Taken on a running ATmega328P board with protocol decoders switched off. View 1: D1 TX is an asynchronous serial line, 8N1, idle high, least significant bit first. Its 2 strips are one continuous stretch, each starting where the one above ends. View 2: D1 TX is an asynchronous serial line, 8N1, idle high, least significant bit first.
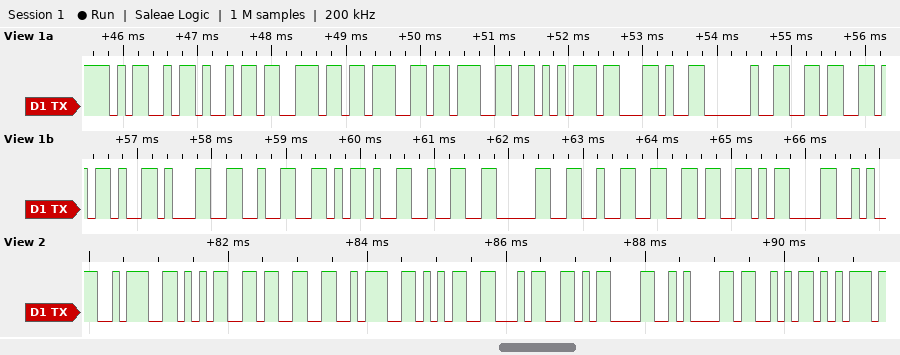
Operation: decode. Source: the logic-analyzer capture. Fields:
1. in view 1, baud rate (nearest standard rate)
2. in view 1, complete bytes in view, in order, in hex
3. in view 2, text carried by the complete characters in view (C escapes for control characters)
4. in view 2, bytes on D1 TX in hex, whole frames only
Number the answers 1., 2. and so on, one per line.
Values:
1. 9600 baud
2. 0x4D 0x69 0x6E 0x67 0x67 0x75 0x2C 0x20 0x36 0x2D 0x31 0x32 0x2D 0x32 0x30 0x32 0x36 0x0D
3. ":53:54\r\nSu"
4. 0x3A 0x35 0x33 0x3A 0x35 0x34 0x0D 0x0A 0x53 0x75
